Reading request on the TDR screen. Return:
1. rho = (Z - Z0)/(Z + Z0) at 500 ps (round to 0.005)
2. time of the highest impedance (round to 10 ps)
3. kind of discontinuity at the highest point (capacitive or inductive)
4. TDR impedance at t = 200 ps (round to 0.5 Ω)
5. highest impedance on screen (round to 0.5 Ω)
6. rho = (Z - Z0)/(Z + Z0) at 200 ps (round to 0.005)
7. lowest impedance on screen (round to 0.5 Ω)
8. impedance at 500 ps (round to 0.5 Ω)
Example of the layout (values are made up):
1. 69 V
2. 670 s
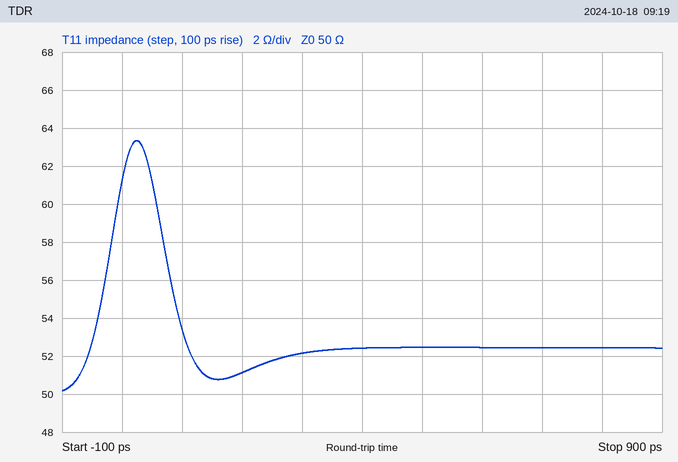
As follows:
1. +0.025
2. 20 ps
3. inductive
4. 51.0 Ω
5. 63.5 Ω
6. +0.010
7. 50.0 Ω
8. 52.5 Ω
